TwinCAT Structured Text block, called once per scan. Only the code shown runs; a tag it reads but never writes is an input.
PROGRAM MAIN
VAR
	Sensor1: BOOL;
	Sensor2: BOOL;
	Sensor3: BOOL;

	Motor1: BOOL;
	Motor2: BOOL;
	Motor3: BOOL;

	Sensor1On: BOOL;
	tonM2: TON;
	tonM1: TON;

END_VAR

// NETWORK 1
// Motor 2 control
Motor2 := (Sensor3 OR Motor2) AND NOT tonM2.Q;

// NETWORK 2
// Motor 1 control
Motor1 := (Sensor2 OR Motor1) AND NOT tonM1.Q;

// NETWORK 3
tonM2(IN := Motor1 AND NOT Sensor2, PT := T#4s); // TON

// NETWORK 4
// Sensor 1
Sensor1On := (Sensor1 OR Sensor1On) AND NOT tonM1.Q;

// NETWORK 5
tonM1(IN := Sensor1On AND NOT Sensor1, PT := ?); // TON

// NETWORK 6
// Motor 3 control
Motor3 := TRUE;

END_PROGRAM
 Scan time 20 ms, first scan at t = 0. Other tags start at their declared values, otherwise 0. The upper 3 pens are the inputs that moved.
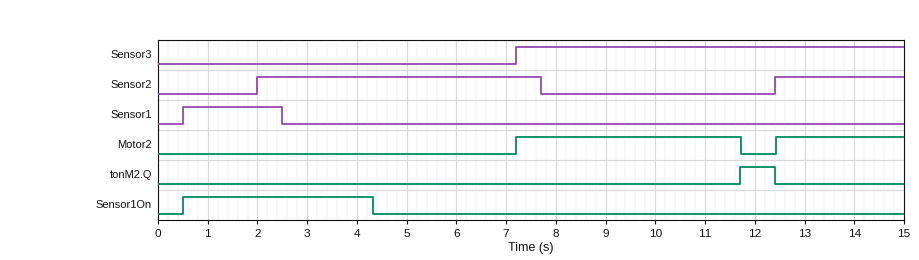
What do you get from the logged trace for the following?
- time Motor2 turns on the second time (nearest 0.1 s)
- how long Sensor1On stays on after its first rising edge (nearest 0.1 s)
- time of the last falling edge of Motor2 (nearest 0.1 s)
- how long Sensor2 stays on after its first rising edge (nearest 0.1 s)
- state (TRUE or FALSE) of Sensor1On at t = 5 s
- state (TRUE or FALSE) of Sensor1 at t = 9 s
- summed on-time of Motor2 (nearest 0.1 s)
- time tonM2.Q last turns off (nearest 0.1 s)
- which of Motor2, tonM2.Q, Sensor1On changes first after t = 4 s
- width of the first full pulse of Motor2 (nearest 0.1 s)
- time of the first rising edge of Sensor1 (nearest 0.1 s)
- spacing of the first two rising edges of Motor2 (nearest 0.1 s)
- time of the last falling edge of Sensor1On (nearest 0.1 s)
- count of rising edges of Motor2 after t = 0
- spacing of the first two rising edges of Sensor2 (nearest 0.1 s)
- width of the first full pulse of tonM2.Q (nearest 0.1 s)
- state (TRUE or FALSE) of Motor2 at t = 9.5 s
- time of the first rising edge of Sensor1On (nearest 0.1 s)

12.4 s
3.8 s
11.7 s
5.7 s
FALSE
FALSE
7.1 s
12.4 s
Sensor1On
4.5 s
0.5 s
5.2 s
4.3 s
2
10.4 s
0.7 s
TRUE
0.5 s
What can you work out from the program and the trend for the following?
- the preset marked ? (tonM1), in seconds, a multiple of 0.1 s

1.8 s
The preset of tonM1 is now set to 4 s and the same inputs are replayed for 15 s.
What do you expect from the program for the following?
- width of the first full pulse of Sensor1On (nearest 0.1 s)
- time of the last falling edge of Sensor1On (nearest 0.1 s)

6.0 s
6.5 s
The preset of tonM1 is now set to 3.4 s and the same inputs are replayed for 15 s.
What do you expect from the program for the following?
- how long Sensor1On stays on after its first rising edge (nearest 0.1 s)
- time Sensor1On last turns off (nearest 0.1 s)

5.4 s
5.9 s
